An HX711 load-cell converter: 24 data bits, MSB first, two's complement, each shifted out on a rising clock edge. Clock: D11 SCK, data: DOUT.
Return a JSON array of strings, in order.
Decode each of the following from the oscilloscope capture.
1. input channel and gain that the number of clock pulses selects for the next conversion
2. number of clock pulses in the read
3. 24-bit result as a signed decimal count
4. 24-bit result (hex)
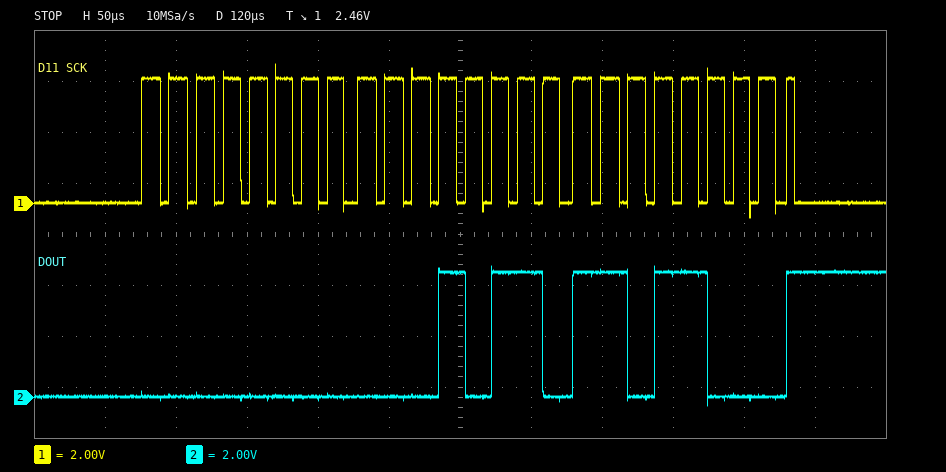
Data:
["channel A, gain 128", "25", "5848", "0x0016D8"]
